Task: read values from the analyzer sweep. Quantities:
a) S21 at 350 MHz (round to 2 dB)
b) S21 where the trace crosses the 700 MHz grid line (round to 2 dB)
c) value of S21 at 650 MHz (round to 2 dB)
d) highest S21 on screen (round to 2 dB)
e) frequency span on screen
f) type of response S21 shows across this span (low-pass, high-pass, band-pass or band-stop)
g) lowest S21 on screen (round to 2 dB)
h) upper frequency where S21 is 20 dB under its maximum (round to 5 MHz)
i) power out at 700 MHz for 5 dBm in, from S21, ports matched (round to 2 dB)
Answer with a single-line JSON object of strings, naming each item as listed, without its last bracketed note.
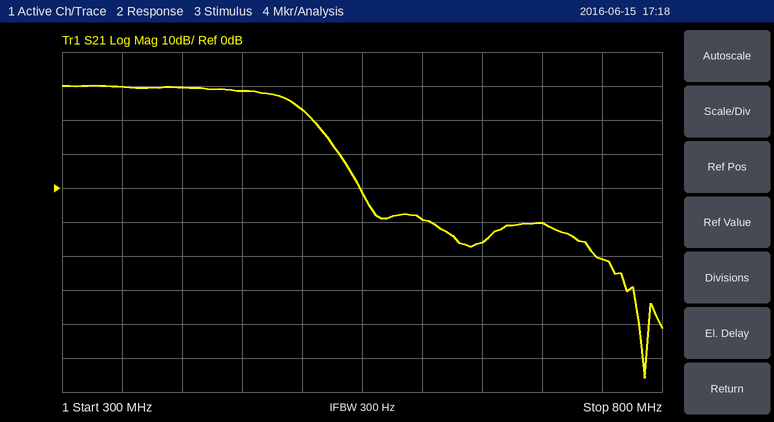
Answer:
{"S21 at 350 MHz": "30 dB", "S21 where the trace crosses the 700 MHz grid line": "-10 dB", "value of S21 at 650 MHz": "-16 dB", "highest S21 on screen": "30 dB", "frequency span on screen": "500 MHz", "type of response S21 shows across this span": "low-pass", "lowest S21 on screen": "-56 dB", "upper frequency where S21 is 20 dB under its maximum": "530 MHz", "power out at 700 MHz for 5 dBm in, from S21, ports matched": "-6 dBm"}
